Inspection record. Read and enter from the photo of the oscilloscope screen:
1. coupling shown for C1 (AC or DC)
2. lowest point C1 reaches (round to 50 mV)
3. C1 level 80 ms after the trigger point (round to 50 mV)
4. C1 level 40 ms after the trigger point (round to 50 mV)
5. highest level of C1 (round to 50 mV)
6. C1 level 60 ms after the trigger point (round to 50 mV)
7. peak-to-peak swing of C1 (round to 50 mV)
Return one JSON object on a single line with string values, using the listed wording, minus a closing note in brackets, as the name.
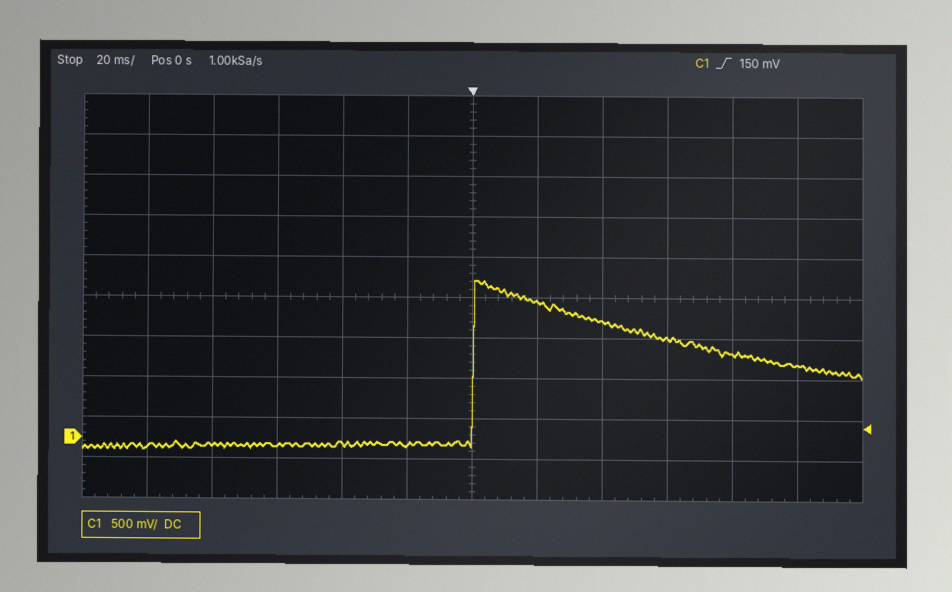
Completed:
{"coupling shown for C1": "DC", "lowest point C1 reaches": "-150 mV", "C1 level 80 ms after the trigger point": "1.05 V", "C1 level 40 ms after the trigger point": "1.45 V", "highest level of C1": "1.95 V", "C1 level 60 ms after the trigger point": "1.25 V", "peak-to-peak swing of C1": "2.10 V"}
